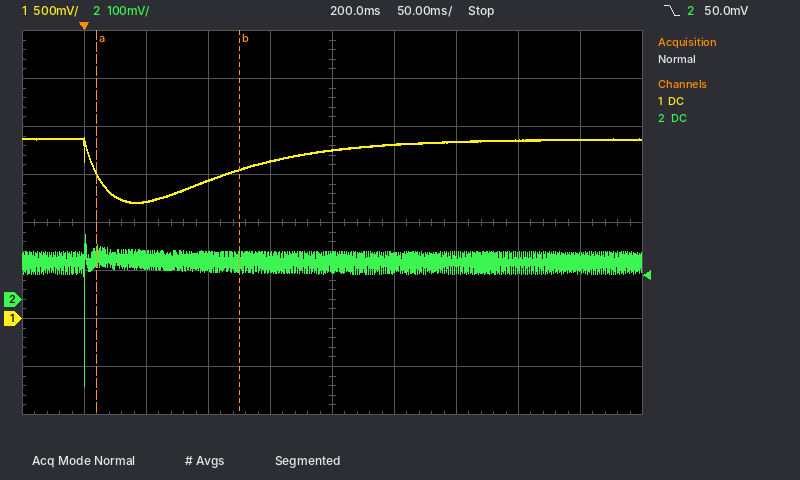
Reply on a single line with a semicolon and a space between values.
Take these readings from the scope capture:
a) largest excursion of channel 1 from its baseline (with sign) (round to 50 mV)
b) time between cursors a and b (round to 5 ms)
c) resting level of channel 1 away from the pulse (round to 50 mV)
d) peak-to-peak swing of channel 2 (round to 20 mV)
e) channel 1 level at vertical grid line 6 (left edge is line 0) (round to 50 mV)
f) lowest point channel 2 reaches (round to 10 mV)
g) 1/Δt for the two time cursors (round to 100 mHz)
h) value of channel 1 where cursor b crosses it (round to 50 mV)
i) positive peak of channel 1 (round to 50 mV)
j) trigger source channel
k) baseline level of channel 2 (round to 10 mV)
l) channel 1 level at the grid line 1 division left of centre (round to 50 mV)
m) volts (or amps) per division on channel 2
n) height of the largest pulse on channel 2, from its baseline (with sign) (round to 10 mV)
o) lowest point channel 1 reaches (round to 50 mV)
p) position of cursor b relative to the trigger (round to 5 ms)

-650 mV; 115 ms; 1.85 V; 320 mV; 1.80 V; -180 mV; 8.7 Hz; 1.55 V; 1.90 V; channel 2; 80 mV; 1.65 V; 100 mV; -260 mV; 1.20 V; +125 ms
